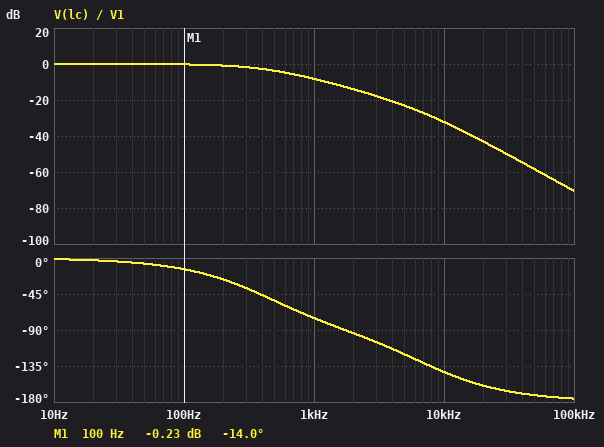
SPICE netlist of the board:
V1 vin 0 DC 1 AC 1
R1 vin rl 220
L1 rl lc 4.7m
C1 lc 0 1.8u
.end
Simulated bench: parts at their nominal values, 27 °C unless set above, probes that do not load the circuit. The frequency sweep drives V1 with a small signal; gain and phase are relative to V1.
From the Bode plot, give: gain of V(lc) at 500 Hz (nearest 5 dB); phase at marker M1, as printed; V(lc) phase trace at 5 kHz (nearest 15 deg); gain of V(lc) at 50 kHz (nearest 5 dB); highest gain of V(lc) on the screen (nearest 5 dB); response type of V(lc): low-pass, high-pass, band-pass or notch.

-5 dB
-14.0 deg
-120 deg
-60 dB
0 dB
low-pass
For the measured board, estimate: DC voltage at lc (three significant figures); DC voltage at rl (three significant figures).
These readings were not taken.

1.00 V
1.00 V
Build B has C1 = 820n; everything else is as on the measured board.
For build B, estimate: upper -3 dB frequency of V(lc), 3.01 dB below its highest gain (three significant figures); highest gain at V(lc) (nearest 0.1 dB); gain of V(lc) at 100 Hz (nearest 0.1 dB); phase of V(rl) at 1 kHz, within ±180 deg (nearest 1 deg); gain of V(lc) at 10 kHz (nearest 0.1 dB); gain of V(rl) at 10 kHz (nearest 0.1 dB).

998 Hz
0 dB
0 dB
-53 deg
-25.2 dB
-2.1 dB
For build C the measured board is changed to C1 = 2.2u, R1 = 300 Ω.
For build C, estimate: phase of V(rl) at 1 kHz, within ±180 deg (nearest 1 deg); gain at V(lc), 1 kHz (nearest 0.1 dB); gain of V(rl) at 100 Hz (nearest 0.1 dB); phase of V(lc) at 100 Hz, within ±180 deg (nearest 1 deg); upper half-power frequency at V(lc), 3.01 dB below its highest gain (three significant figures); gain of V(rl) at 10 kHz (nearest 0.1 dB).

-82 deg
-12.4 dB
-0.7 dB
-23 deg
247 Hz
-3.2 dB
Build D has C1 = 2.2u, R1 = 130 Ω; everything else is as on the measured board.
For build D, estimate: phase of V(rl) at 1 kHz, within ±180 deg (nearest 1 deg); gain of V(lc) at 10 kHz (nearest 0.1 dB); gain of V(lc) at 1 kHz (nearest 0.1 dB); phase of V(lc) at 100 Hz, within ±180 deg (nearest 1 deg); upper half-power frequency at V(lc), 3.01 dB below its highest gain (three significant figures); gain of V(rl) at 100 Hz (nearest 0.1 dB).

-72 deg
-32.8 dB
-5.5 dB
-10 deg
635 Hz
-0.1 dB
